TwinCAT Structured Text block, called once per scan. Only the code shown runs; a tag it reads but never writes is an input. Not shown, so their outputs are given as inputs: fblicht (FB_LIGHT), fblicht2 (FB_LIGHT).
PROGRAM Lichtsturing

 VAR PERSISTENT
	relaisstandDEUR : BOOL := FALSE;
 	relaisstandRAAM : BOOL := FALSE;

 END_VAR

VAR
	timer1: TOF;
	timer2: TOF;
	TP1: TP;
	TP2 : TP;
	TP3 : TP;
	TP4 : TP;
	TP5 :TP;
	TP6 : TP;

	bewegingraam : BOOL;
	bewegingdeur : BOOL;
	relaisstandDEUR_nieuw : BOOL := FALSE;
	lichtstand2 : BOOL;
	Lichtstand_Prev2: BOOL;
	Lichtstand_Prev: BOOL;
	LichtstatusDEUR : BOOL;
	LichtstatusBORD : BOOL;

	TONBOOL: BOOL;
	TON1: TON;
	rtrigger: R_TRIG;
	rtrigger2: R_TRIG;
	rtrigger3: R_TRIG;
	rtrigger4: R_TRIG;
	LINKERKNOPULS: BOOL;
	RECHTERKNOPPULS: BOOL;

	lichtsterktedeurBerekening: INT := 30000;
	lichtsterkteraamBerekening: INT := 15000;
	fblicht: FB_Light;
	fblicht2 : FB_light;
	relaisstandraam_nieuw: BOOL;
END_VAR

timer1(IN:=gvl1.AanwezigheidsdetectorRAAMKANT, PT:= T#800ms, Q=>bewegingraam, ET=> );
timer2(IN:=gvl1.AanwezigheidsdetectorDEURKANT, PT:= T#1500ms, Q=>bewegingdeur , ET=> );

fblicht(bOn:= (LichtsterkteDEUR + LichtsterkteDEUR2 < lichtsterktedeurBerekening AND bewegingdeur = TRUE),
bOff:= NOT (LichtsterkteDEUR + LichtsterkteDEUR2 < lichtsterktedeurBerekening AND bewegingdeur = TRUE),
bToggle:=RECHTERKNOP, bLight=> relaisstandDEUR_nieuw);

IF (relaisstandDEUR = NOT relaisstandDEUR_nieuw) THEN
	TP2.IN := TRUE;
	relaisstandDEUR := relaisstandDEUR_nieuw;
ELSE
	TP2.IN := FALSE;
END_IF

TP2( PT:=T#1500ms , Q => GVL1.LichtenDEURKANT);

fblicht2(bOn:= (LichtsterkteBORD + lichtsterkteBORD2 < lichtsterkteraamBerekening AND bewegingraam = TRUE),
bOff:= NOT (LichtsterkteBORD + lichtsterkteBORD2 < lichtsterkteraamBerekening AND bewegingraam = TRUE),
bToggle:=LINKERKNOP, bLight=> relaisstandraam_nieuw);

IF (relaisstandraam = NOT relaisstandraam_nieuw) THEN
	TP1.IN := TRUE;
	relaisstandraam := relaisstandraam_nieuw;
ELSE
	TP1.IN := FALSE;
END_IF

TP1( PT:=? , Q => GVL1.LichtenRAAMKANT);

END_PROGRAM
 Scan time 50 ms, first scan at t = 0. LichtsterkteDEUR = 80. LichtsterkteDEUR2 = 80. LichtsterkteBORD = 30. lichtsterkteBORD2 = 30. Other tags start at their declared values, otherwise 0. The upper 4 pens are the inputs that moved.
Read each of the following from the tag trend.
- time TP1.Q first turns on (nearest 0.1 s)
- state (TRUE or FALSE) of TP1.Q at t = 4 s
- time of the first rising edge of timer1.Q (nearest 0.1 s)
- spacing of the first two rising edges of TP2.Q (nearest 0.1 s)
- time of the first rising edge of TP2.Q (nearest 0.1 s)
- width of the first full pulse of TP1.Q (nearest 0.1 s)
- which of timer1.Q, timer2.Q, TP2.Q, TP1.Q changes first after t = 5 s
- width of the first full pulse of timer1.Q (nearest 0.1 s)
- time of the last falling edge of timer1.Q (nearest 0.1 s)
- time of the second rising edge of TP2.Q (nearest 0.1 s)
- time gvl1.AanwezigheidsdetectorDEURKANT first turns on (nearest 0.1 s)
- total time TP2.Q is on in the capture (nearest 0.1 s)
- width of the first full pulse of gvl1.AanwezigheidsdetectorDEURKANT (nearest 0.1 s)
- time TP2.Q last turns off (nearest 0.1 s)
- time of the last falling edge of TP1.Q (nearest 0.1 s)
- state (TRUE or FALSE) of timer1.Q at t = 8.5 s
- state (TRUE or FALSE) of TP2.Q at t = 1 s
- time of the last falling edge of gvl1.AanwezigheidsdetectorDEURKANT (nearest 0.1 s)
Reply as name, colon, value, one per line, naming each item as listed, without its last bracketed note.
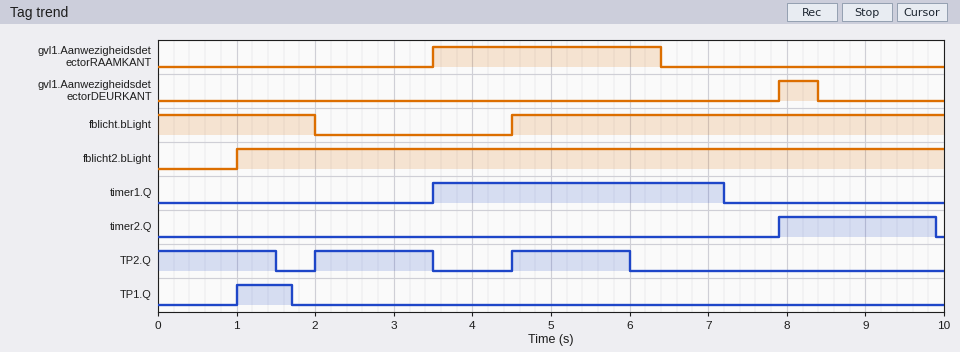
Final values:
time TP1.Q first turns on: 1.0 s
state (TRUE or FALSE) of TP1.Q at t = 4 s: FALSE
time of the first rising edge of timer1.Q: 3.5 s
spacing of the first two rising edges of TP2.Q: 2.5 s
time of the first rising edge of TP2.Q: 2.0 s
width of the first full pulse of TP1.Q: 0.7 s
which of timer1.Q, timer2.Q, TP2.Q, TP1.Q changes first after t = 5 s: TP2.Q
width of the first full pulse of timer1.Q: 3.7 s
time of the last falling edge of timer1.Q: 7.2 s
time of the second rising edge of TP2.Q: 4.5 s
time gvl1.AanwezigheidsdetectorDEURKANT first turns on: 7.9 s
total time TP2.Q is on in the capture: 4.5 s
width of the first full pulse of gvl1.AanwezigheidsdetectorDEURKANT: 0.5 s
time TP2.Q last turns off: 6.0 s
time of the last falling edge of TP1.Q: 1.7 s
state (TRUE or FALSE) of timer1.Q at t = 8.5 s: FALSE
state (TRUE or FALSE) of TP2.Q at t = 1 s: TRUE
time of the last falling edge of gvl1.AanwezigheidsdetectorDEURKANT: 8.4 s
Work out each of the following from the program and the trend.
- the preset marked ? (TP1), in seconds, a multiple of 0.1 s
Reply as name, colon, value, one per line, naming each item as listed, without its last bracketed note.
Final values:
the preset marked ? (TP1), in seconds, a multiple of 0.1 s: 0.7 s
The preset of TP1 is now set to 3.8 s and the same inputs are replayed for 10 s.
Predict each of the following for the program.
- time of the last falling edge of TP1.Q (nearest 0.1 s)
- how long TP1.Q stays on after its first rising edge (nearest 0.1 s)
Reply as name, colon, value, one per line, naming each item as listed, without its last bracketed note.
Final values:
time of the last falling edge of TP1.Q: 4.8 s
how long TP1.Q stays on after its first rising edge: 3.8 s
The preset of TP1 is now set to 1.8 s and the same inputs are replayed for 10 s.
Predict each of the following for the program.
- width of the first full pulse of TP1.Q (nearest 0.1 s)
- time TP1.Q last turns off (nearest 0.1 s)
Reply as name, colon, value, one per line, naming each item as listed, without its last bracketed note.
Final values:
width of the first full pulse of TP1.Q: 1.8 s
time TP1.Q last turns off: 2.8 s
